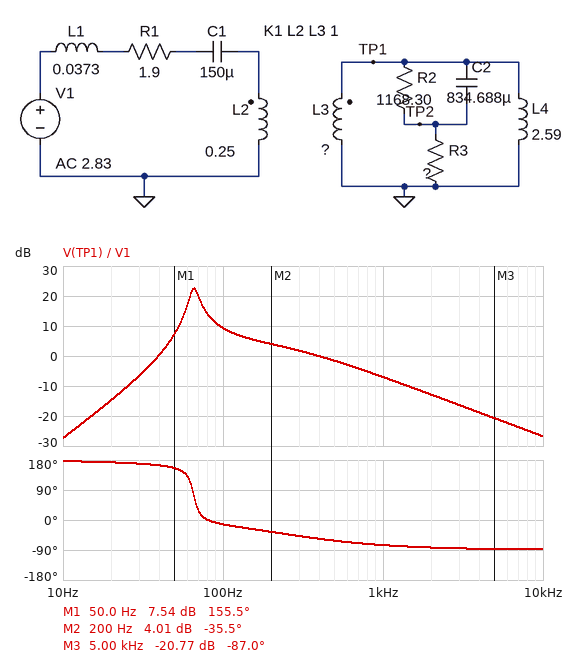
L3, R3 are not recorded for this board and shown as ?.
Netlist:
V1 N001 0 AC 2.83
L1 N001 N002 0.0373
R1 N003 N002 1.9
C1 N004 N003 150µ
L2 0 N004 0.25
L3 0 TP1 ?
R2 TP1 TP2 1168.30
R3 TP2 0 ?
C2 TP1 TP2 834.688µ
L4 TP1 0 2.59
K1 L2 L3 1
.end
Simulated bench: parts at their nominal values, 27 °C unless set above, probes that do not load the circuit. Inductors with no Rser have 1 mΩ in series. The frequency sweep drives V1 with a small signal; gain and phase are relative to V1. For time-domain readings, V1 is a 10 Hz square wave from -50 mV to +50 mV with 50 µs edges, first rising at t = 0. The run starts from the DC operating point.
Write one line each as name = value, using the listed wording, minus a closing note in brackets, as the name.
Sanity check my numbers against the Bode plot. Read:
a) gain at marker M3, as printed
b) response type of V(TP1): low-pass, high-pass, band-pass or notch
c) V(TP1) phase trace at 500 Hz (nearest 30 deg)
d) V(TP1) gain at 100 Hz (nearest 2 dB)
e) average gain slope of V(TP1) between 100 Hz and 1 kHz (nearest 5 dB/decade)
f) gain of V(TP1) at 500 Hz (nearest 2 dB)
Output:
gain at marker M3, as printed = -20.77 dB
response type of V(TP1): low-pass, high-pass, band-pass or notch = band-pass
V(TP1) phase trace at 500 Hz = -60 deg
V(TP1) gain at 100 Hz = 10 dB
average gain slope of V(TP1) between 100 Hz and 1 kHz = -15 dB/decade
gain of V(TP1) at 500 Hz = -2 dB
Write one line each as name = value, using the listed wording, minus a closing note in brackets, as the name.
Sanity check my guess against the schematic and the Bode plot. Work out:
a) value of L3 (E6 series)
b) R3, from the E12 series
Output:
value of L3 = 330 H
R3, from the E12 series = 3.9 kΩ
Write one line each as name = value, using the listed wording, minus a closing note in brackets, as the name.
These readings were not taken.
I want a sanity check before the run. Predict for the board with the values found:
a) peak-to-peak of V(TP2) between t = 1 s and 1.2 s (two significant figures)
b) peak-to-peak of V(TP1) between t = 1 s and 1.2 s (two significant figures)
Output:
peak-to-peak of V(TP2) between t = 1 s and 1.2 s = 310 mV
peak-to-peak of V(TP1) between t = 1 s and 1.2 s = 310 mV
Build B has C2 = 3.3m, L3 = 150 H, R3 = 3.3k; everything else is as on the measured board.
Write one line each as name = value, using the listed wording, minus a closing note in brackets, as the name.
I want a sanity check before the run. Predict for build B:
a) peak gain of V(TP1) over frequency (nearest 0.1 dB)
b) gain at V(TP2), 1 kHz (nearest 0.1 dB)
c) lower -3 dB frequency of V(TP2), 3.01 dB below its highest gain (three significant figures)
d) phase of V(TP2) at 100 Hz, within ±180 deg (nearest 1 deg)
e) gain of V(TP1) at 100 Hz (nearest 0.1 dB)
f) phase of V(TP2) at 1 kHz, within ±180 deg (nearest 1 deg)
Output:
peak gain of V(TP1) over frequency = 24.5 dB
gain at V(TP2), 1 kHz = -5.0 dB
lower -3 dB frequency of V(TP2), 3.01 dB below its highest gain = 60.0 Hz
phase of V(TP2) at 100 Hz, within ±180 deg = -15 deg
gain of V(TP1) at 100 Hz = 11.7 dB
phase of V(TP2) at 1 kHz, within ±180 deg = -77 deg
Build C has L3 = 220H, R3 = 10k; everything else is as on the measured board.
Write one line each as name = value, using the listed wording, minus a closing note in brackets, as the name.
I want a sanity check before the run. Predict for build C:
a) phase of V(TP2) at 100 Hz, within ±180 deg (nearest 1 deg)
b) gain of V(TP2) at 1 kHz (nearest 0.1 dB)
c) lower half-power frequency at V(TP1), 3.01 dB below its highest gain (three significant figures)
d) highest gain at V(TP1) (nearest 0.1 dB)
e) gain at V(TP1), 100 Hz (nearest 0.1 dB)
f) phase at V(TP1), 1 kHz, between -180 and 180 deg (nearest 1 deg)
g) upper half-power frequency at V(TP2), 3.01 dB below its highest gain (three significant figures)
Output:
phase of V(TP2) at 100 Hz, within ±180 deg = -1 deg
gain of V(TP2) at 1 kHz = 1.6 dB
lower half-power frequency at V(TP1), 3.01 dB below its highest gain = 61.3 Hz
highest gain at V(TP1) = 24.8 dB
gain at V(TP1), 100 Hz = 11.2 dB
phase at V(TP1), 1 kHz, between -180 and 180 deg = -56 deg
upper half-power frequency at V(TP2), 3.01 dB below its highest gain = 69.5 Hz
